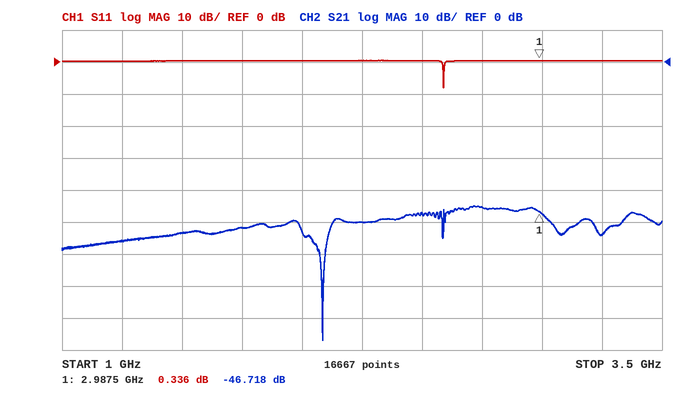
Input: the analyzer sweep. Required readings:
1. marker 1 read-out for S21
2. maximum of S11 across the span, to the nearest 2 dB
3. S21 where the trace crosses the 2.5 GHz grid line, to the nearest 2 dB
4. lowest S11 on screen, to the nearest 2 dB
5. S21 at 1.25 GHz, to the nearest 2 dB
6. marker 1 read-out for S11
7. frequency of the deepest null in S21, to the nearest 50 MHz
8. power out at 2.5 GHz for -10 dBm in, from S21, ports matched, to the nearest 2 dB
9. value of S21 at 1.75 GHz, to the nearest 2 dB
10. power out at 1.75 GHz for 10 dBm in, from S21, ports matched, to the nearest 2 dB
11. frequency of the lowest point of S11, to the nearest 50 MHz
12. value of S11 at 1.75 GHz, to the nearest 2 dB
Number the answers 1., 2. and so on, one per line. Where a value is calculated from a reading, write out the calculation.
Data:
1. -46.718 dB
2. 0 dB
3. -48 dB
4. -8 dB
5. -56 dB
6. 0.336 dB
7. 2.10 GHz
8. -10 dBm + (-48 dB) = -58 dBm
9. -52 dB
10. 10 dBm + (-52 dB) = -42 dBm
11. 2.60 GHz
12. 0 dB
